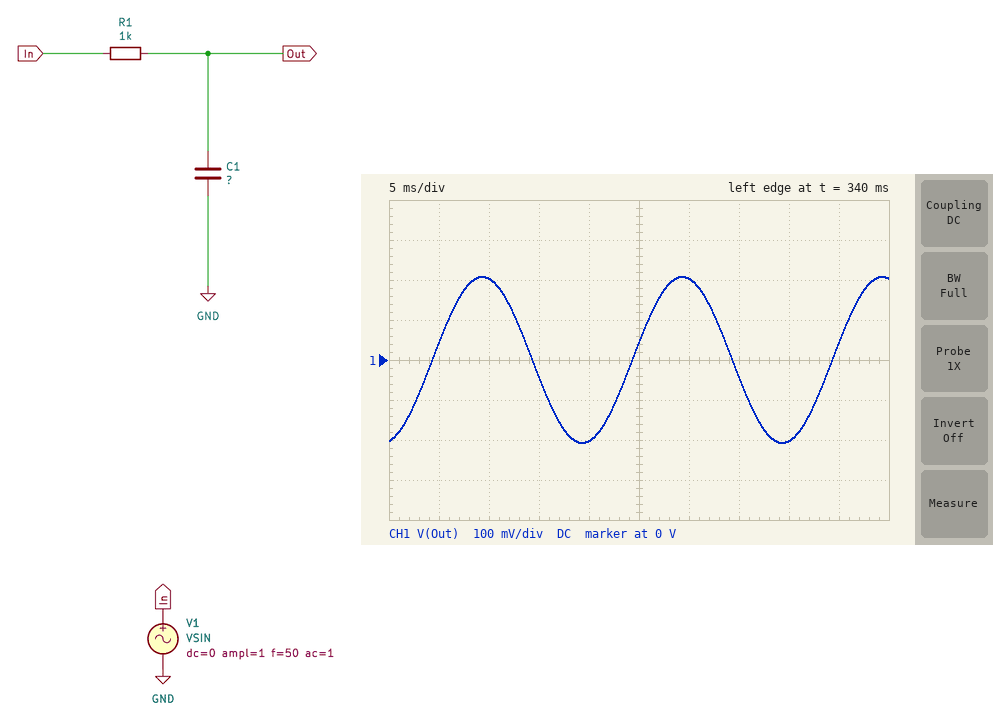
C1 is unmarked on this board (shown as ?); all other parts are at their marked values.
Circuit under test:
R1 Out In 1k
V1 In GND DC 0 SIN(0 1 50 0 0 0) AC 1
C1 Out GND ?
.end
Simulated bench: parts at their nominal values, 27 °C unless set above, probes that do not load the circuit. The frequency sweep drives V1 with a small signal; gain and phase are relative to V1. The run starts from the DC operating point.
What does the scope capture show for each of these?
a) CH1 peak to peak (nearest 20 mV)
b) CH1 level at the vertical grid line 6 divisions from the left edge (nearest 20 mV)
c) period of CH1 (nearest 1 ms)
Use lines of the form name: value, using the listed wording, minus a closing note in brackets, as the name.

CH1 peak to peak: 420 mV
CH1 level at the vertical grid line 6 divisions from the left edge: 200 mV
period of CH1: 20 ms
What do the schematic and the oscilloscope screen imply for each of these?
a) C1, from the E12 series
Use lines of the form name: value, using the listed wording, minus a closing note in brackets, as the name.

C1, from the E12 series: 15 µF
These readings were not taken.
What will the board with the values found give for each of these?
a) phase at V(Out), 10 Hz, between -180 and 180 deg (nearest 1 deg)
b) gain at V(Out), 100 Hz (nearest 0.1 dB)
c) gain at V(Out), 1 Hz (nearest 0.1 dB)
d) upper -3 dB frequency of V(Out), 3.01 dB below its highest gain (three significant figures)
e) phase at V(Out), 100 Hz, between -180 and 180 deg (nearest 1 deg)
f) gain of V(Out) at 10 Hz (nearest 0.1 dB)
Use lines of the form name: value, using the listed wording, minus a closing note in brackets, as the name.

phase at V(Out), 10 Hz, between -180 and 180 deg: -43 deg
gain at V(Out), 100 Hz: -19.5 dB
gain at V(Out), 1 Hz: 0 dB
upper -3 dB frequency of V(Out), 3.01 dB below its highest gain: 10.6 Hz
phase at V(Out), 100 Hz, between -180 and 180 deg: -84 deg
gain of V(Out) at 10 Hz: -2.8 dB
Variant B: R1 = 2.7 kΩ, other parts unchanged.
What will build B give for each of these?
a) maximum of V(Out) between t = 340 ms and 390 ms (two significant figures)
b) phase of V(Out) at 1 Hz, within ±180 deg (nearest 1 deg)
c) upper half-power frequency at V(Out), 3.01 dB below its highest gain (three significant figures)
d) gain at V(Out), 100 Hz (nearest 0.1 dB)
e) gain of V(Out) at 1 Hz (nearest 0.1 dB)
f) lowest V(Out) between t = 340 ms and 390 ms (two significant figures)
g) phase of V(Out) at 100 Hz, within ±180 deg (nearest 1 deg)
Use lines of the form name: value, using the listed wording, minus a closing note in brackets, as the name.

maximum of V(Out) between t = 340 ms and 390 ms: 78 mV
phase of V(Out) at 1 Hz, within ±180 deg: -14 deg
upper half-power frequency at V(Out), 3.01 dB below its highest gain: 3.93 Hz
gain at V(Out), 100 Hz: -28.1 dB
gain of V(Out) at 1 Hz: -0.3 dB
lowest V(Out) between t = 340 ms and 390 ms: -78 mV
phase of V(Out) at 100 Hz, within ±180 deg: -88 deg
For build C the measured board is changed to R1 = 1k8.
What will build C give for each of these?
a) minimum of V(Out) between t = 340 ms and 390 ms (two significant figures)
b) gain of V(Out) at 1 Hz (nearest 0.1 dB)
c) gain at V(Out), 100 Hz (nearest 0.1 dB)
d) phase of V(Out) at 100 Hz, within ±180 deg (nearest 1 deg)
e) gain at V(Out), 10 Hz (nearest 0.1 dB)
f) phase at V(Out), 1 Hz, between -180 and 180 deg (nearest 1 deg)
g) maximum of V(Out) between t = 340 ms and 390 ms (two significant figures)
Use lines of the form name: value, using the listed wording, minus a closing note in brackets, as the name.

minimum of V(Out) between t = 340 ms and 390 ms: -120 mV
gain of V(Out) at 1 Hz: -0.1 dB
gain at V(Out), 100 Hz: -24.6 dB
phase of V(Out) at 100 Hz, within ±180 deg: -87 deg
gain at V(Out), 10 Hz: -5.9 dB
phase at V(Out), 1 Hz, between -180 and 180 deg: -10 deg
maximum of V(Out) between t = 340 ms and 390 ms: 120 mV
